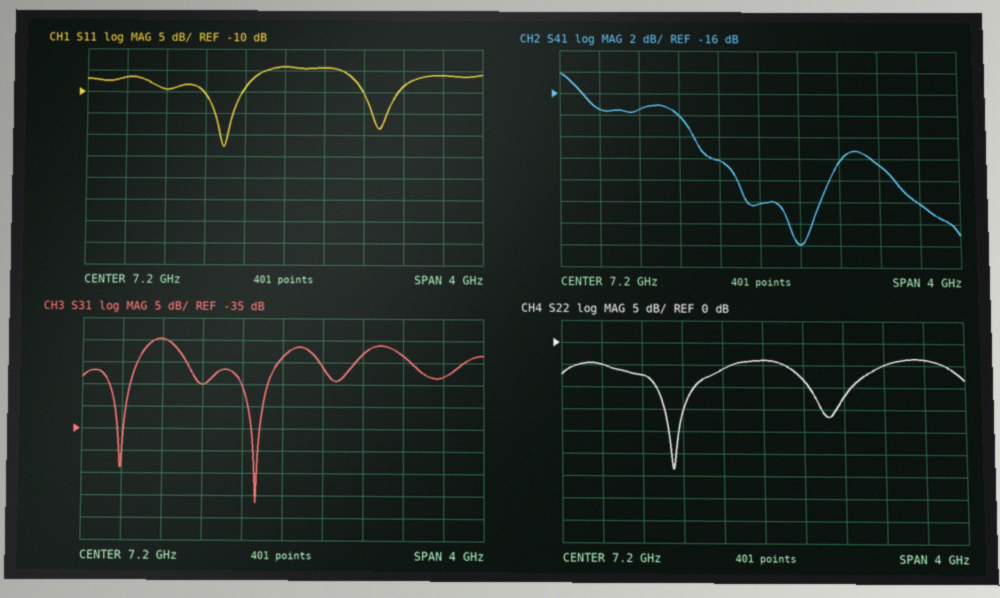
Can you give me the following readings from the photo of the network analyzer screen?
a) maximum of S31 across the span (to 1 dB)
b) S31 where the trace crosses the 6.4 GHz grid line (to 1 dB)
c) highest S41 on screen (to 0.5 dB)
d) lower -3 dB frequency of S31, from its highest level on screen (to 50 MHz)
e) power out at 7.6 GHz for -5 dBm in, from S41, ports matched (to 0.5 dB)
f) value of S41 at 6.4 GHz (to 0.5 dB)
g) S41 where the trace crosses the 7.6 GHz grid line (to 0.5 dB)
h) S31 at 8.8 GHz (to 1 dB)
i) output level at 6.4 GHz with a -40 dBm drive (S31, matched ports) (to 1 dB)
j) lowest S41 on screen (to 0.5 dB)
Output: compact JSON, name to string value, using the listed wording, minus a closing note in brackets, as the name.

{"maximum of S31 across the span": "-15 dB", "S31 where the trace crosses the 6.4 GHz grid line": "-25 dB", "highest S41 on screen": "-14.0 dB", "lower -3 dB frequency of S31, from its highest level on screen": "5.80 GHz", "power out at 7.6 GHz for -5 dBm in, from S41, ports matched": "-35.0 dBm", "value of S41 at 6.4 GHz": "-18.0 dB", "S41 where the trace crosses the 7.6 GHz grid line": "-30.0 dB", "S31 at 8.8 GHz": "-23 dB", "output level at 6.4 GHz with a -40 dBm drive (S31, matched ports)": "-65 dBm", "lowest S41 on screen": "-30.0 dB"}
